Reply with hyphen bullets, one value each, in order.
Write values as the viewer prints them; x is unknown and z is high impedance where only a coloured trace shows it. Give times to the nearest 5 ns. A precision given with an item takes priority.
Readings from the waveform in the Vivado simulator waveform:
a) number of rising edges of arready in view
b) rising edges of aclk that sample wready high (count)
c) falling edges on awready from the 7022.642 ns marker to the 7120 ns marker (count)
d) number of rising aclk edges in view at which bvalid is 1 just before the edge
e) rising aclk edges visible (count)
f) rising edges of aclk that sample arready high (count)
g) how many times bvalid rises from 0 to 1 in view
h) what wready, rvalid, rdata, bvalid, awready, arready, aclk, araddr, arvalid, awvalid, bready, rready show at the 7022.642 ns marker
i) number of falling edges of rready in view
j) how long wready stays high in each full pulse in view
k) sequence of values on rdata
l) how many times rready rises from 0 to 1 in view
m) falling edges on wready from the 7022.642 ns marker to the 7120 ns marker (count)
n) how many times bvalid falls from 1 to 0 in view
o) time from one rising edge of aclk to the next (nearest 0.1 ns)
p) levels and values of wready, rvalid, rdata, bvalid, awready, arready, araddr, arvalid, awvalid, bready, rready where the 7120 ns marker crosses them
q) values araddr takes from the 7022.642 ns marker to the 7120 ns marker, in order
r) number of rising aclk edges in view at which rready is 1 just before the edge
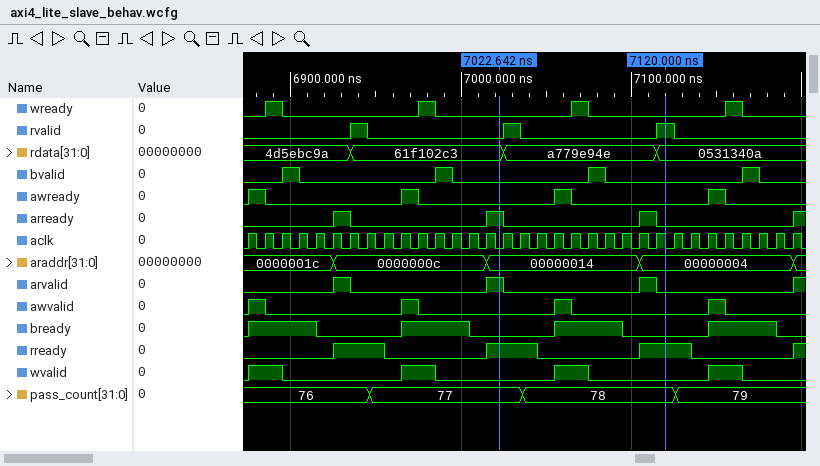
- 4
- 4
- 1
- 4
- 33
- 3
- 4
- wready=0, rvalid=0, rdata=61f102c3, bvalid=0, awready=0, arready=1, aclk=0, araddr=00000014, arvalid=1, awvalid=0, bready=0, rready=1
- 3
- 10 ns, 10 ns, 10 ns, 10 ns
- 4d5ebc9a, 61f102c3, a779e94e, 0531340a
- 4
- 1
- 4
- 10 ns
- wready=0, rvalid=1, rdata=0531340a, bvalid=0, awready=0, arready=0, araddr=00000004, arvalid=0, awvalid=0, bready=0, rready=1
- 00000014, 00000004
- 9
